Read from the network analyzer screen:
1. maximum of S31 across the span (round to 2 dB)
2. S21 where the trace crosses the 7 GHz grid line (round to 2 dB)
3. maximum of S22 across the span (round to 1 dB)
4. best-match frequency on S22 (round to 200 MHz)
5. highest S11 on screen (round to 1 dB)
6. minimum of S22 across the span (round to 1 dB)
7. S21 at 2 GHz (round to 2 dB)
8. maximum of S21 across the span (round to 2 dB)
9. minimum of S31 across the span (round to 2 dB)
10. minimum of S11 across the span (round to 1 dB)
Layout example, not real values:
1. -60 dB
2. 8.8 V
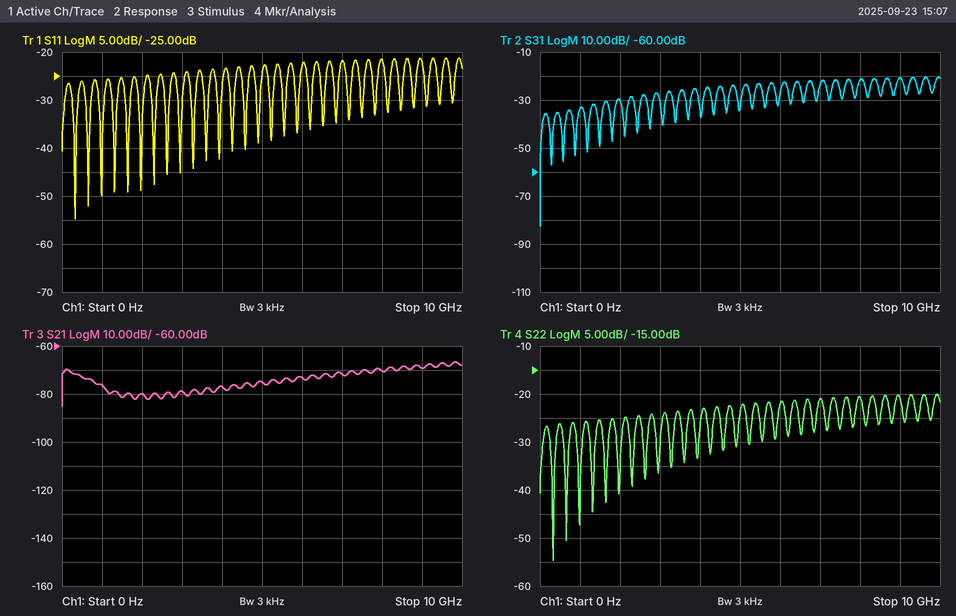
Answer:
1. -20 dB
2. -72 dB
3. -20 dB
4. 400 MHz
5. -21 dB
6. -55 dB
7. -80 dB
8. -66 dB
9. -82 dB
10. -55 dB
